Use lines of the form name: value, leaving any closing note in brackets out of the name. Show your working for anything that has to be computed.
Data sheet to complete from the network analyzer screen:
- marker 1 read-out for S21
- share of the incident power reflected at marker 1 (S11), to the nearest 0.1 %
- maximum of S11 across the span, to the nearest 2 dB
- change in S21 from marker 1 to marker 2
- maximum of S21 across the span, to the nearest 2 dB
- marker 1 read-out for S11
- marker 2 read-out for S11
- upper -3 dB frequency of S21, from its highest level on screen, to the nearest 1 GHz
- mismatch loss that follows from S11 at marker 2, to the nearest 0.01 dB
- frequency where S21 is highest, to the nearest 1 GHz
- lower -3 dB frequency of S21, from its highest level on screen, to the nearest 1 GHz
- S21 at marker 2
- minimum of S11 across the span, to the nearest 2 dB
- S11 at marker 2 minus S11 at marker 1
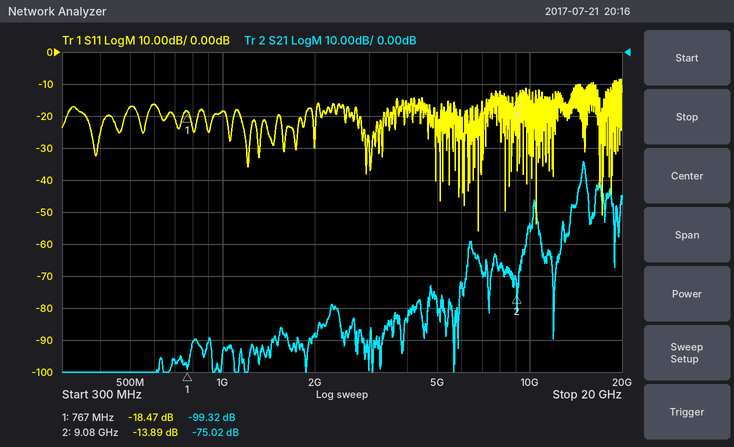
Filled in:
marker 1 read-out for S21: -99.32 dB
share of the incident power reflected at marker 1 (S11), to the nearest 0.1 %: 10^(-18.47/10) ≈ 1.4 %
maximum of S11 across the span, to the nearest 2 dB: -8 dB
change in S21 from marker 1 to marker 2: -75.02 − (-99.32) = 24.30 dB
maximum of S21 across the span, to the nearest 2 dB: -34 dB
marker 1 read-out for S11: -18.47 dB
marker 2 read-out for S11: -13.89 dB
upper -3 dB frequency of S21, from its highest level on screen, to the nearest 1 GHz: 15 GHz
mismatch loss that follows from S11 at marker 2, to the nearest 0.01 dB: −10 log10(1 − 10^(-13.89/10)) ≈ 0.18 dB
frequency where S21 is highest, to the nearest 1 GHz: 15 GHz
lower -3 dB frequency of S21, from its highest level on screen, to the nearest 1 GHz: 15 GHz
S21 at marker 2: -75.02 dB
minimum of S11 across the span, to the nearest 2 dB: -56 dB
S11 at marker 2 minus S11 at marker 1: -13.89 − (-18.47) = 4.58 dB
